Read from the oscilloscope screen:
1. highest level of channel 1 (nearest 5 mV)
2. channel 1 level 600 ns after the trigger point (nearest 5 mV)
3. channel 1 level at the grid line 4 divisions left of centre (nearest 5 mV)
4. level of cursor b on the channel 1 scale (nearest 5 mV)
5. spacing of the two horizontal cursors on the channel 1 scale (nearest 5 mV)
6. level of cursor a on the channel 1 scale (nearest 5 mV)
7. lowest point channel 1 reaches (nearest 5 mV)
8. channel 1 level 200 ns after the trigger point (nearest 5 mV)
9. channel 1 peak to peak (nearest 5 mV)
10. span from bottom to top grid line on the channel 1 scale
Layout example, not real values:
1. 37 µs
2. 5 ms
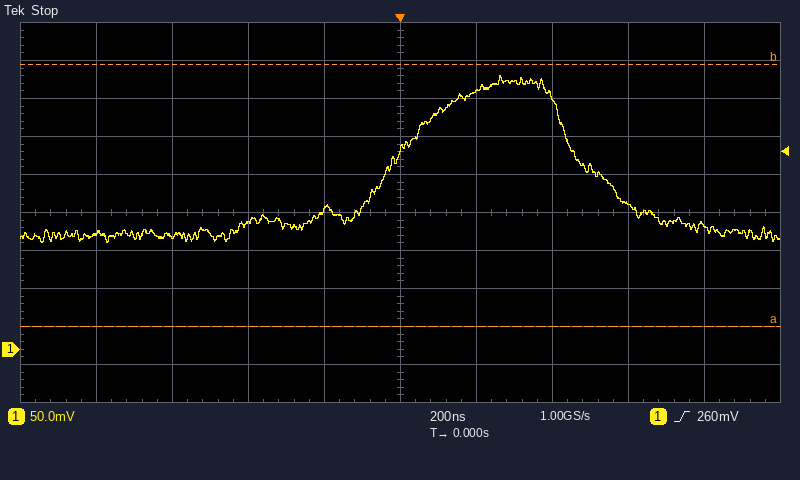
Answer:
1. 360 mV
2. 190 mV
3. 150 mV
4. 375 mV
5. 345 mV
6. 30 mV
7. 140 mV
8. 340 mV
9. 220 mV
10. 500 mV
